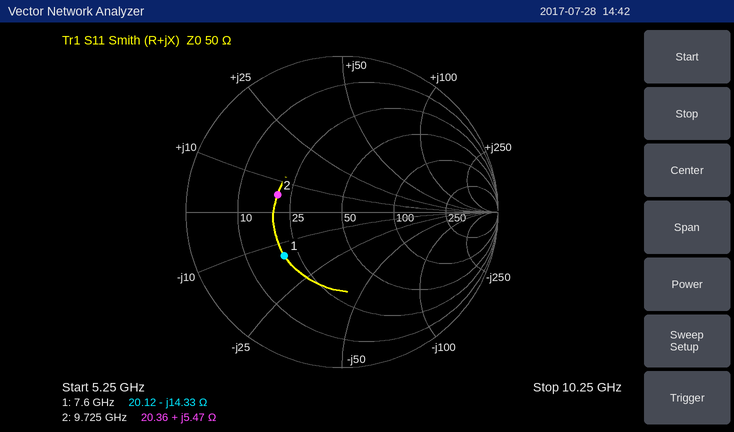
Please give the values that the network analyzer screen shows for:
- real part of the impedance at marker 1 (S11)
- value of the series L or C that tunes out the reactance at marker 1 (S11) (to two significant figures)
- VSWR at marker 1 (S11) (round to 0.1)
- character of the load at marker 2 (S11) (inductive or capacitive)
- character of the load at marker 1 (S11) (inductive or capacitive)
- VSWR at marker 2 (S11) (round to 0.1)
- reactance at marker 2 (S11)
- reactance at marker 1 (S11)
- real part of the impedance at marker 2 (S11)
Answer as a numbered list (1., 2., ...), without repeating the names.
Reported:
1. 20.12 Ω
2. 300 pH
3. 2.7
4. inductive
5. capacitive
6. 2.5
7. +5.47 Ω
8. -14.33 Ω
9. 20.36 Ω
